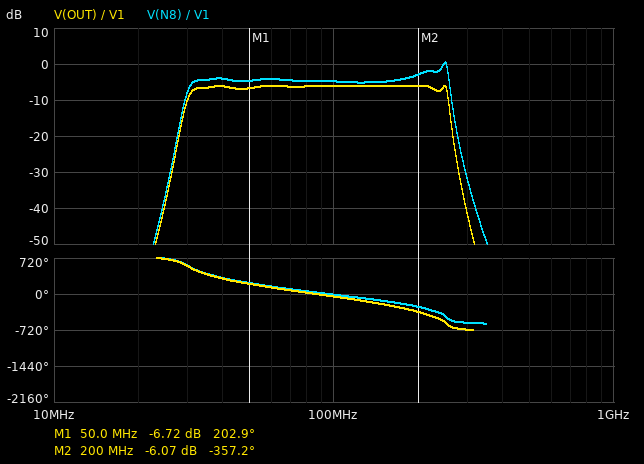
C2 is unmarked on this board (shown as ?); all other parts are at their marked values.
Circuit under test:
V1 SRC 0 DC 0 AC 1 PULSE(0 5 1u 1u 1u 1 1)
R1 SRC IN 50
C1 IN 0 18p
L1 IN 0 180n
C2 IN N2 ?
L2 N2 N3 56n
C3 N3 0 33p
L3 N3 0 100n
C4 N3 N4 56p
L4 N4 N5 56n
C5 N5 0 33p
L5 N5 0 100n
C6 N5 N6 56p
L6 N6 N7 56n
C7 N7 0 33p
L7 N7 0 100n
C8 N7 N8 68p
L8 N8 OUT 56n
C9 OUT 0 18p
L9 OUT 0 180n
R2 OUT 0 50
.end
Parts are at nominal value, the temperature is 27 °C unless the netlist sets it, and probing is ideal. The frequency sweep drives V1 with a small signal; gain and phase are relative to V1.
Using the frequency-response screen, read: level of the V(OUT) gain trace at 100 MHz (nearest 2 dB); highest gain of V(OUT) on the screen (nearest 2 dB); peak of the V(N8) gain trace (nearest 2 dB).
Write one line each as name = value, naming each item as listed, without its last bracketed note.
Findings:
level of the V(OUT) gain trace at 100 MHz = -6 dB
highest gain of V(OUT) on the screen = -6 dB
peak of the V(N8) gain trace = 0 dB
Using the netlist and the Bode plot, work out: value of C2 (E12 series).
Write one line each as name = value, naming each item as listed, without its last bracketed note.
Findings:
value of C2 = 82 pF
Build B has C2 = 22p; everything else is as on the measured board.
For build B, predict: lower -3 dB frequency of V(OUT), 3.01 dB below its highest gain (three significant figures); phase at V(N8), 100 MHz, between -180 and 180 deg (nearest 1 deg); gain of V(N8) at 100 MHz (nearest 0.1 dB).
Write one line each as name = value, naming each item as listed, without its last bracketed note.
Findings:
lower -3 dB frequency of V(OUT), 3.01 dB below its highest gain = 48.7 MHz
phase at V(N8), 100 MHz, between -180 and 180 deg = 15 deg
gain of V(N8) at 100 MHz = -6.2 dB
